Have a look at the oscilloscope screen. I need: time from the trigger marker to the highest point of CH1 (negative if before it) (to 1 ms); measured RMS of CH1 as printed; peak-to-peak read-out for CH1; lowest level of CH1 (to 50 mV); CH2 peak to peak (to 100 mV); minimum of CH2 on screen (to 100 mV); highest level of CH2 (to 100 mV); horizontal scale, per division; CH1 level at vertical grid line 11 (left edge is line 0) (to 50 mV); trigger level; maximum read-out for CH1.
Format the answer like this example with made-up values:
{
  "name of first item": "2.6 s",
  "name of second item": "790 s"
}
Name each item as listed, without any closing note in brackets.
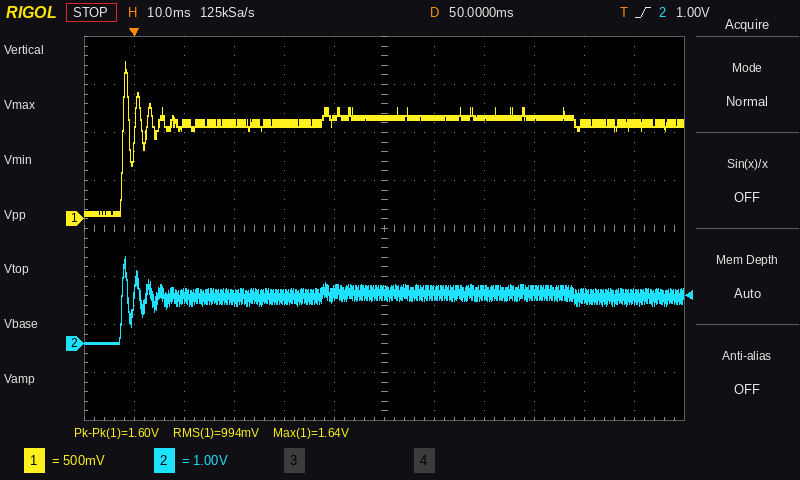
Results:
{
  "time from the trigger marker to the highest point of CH1 (negative if before it)": "-2 ms",
  "measured RMS of CH1 as printed": "994 mV",
  "peak-to-peak read-out for CH1": "1.60 V",
  "lowest level of CH1": "50 mV",
  "CH2 peak to peak": "1.8 V",
  "minimum of CH2 on screen": "0.0 V",
  "highest level of CH2": "1.8 V",
  "horizontal scale, per division": "10 ms",
  "CH1 level at vertical grid line 11 (left edge is line 0)": "1.00 V",
  "trigger level": "1.00 V",
  "maximum read-out for CH1": "1.64 V"
}
